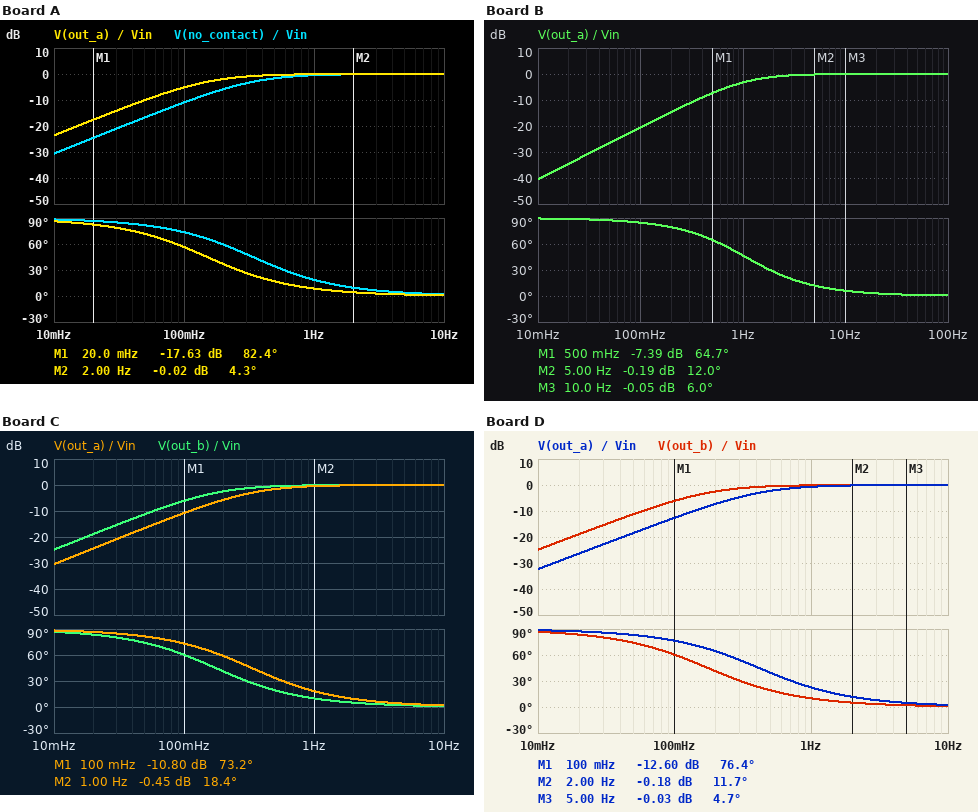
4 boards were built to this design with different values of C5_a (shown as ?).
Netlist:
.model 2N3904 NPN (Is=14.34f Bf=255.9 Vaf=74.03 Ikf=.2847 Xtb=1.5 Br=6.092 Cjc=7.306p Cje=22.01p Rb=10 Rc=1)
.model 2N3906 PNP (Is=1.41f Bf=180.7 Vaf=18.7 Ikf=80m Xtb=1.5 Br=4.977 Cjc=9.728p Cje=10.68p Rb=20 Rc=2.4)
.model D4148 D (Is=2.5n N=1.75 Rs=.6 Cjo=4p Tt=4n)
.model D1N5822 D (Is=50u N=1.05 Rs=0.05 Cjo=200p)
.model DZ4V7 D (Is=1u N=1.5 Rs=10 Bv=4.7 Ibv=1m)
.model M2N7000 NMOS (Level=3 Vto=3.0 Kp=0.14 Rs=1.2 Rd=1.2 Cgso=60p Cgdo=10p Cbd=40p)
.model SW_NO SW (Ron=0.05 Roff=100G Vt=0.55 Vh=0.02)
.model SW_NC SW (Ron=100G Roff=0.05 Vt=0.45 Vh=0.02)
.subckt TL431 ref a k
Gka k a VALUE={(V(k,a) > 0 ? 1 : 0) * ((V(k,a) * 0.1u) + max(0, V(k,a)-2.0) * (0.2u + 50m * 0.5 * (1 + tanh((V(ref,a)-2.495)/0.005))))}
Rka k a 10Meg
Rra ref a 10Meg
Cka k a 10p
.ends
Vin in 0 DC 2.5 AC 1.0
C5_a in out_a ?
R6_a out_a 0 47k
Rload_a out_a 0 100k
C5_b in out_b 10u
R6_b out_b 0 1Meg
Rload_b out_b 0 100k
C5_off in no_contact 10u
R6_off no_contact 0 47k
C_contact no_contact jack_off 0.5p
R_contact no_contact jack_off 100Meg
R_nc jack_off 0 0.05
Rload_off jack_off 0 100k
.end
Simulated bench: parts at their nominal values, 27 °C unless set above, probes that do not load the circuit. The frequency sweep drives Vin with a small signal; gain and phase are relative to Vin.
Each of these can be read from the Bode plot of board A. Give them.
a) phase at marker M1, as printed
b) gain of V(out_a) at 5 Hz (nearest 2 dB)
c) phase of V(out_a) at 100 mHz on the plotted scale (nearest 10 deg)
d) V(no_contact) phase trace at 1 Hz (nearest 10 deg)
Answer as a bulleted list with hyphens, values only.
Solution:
- 82.4 deg
- 0 dB
- 60 deg
- 20 deg
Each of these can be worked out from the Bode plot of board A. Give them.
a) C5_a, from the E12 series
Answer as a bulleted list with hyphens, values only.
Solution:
- 33 µF
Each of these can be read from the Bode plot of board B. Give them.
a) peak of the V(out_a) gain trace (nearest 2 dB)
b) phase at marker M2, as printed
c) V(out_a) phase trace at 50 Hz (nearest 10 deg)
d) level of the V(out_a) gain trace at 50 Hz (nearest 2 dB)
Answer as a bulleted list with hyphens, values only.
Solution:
- 0 dB
- 12.0 deg
- 0 deg
- 0 dB
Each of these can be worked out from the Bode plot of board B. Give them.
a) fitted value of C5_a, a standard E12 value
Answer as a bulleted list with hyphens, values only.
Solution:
- 4.7 µF
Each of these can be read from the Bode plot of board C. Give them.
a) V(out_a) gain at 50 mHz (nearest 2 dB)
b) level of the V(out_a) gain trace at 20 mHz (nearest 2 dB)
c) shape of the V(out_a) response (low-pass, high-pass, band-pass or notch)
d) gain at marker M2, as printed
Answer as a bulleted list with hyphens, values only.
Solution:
- -16 dB
- -24 dB
- high-pass
- -0.45 dB
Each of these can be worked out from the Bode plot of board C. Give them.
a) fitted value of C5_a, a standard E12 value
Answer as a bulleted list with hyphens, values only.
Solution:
- 15 µF
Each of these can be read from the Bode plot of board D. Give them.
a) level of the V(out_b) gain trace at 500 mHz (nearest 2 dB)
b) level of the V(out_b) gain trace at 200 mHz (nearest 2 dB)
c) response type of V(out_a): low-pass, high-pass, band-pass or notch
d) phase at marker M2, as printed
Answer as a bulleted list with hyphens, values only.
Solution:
- 0 dB
- -2 dB
- high-pass
- 11.7 deg
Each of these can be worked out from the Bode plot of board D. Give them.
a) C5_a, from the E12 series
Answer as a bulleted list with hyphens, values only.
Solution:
- 12 µF
